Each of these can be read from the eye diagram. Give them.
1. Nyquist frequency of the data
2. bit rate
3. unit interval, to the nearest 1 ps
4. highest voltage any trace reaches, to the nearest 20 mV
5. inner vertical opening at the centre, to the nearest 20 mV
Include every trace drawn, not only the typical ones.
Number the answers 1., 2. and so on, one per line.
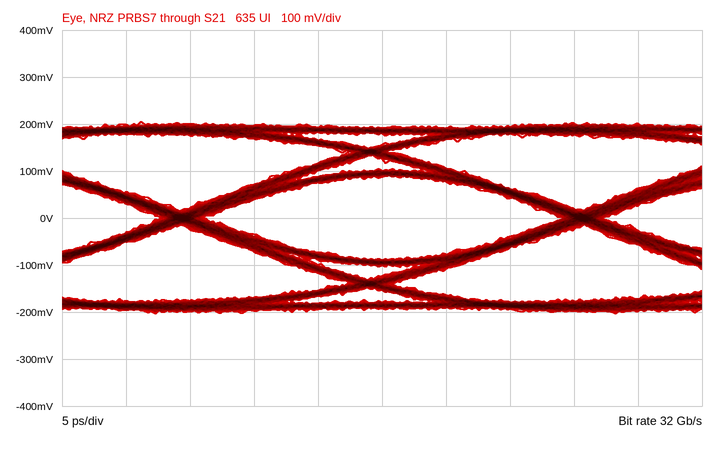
1. 16 GHz
2. 32 Gb/s
3. 31 ps
4. 200 mV
5. 180 mV
